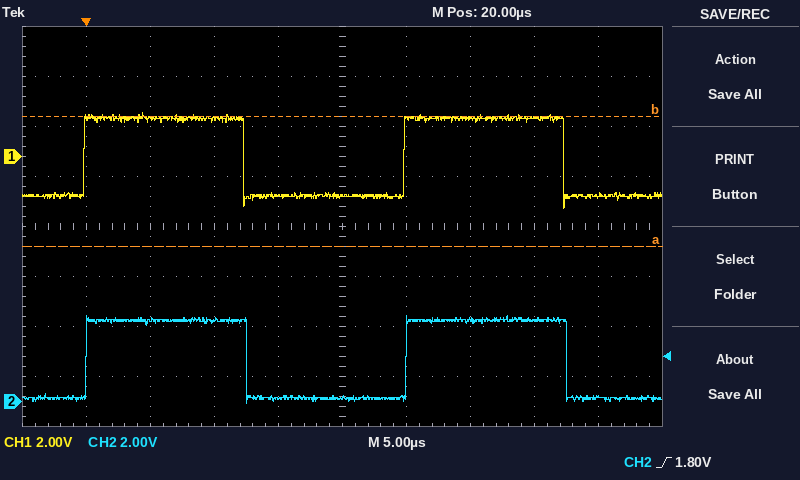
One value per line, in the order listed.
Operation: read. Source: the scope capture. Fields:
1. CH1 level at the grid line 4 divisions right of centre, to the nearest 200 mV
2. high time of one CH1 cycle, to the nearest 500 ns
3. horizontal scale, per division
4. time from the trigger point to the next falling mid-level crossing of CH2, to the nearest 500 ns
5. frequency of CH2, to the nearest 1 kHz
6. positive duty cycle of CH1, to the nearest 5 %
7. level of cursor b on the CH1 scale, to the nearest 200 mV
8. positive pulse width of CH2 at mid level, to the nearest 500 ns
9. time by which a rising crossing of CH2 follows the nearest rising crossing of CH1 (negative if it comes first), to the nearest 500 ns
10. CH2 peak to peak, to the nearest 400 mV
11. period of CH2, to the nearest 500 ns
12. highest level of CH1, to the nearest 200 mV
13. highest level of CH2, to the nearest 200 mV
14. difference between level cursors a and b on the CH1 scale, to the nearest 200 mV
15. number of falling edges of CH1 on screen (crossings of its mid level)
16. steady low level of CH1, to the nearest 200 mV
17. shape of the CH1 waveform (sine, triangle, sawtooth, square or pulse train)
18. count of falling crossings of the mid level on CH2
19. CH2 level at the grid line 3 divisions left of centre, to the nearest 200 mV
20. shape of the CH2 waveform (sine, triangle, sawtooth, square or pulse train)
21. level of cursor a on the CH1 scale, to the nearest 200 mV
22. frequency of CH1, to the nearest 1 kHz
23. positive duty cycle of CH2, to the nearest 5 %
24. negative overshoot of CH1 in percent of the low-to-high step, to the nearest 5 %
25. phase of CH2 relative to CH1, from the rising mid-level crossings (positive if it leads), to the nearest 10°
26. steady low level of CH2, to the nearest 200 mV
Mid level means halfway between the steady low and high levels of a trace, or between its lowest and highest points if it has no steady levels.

-1.6 V
12.5 µs
5 µs
12.5 µs
40 kHz
50 %
1.6 V
12.5 µs
0.0 µs
3.6 V
25.0 µs
1.8 V
3.4 V
5.2 V
2
-1.6 V
square
2
3.2 V
square
-3.6 V
40 kHz
50 %
15 %
0°
200 mV
